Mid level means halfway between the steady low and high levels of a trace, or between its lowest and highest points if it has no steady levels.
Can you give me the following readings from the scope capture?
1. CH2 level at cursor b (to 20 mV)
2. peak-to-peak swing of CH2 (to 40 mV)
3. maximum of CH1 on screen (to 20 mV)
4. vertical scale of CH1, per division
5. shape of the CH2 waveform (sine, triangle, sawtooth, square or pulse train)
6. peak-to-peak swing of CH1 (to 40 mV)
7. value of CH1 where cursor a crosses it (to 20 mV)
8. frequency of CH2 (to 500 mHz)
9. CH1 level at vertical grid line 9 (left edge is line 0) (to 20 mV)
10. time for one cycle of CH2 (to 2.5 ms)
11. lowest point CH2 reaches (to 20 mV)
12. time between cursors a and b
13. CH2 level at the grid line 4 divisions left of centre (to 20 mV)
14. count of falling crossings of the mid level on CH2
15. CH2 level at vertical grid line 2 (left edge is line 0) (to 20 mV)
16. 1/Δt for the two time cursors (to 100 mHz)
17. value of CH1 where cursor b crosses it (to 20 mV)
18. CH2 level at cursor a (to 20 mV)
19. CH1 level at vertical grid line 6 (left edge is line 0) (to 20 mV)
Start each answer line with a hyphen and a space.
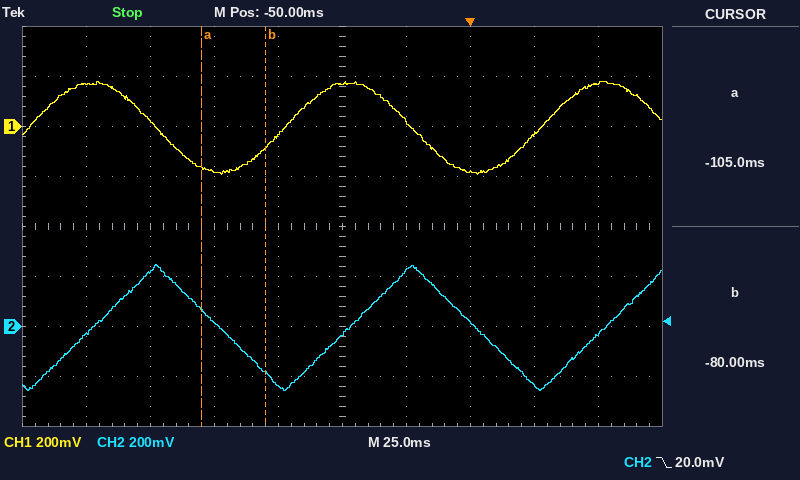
- -180 mV
- 520 mV
- 180 mV
- 200 mV
- triangle
- 360 mV
- -160 mV
- 10.0 Hz
- 180 mV
- 100.0 ms
- -260 mV
- 25.0 ms
- -20 mV
- 2
- 220 mV
- 40.0 Hz
- -80 mV
- 60 mV
- 20 mV
